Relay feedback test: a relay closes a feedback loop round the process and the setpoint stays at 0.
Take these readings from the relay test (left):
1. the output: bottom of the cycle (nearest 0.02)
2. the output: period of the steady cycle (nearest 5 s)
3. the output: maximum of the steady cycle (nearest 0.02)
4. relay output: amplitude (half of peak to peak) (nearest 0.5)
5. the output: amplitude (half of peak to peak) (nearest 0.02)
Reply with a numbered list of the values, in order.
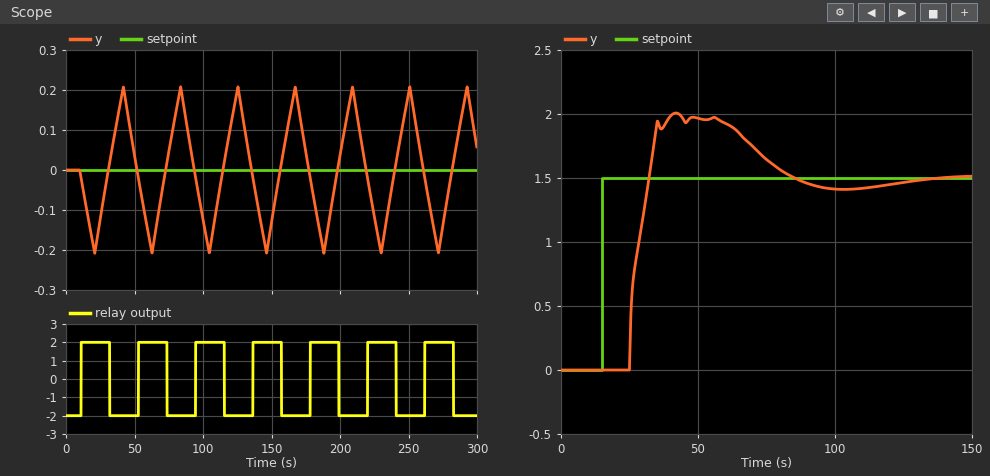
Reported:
1. -0.20
2. 40 s
3. 0.20
4. 2.0
5. 0.20
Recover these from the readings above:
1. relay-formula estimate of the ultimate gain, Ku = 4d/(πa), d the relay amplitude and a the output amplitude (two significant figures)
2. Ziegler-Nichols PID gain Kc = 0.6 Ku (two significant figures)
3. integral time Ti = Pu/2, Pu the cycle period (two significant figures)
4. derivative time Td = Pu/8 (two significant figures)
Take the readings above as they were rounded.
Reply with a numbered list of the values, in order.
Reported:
1. 13
2. 7.8
3. 20 s
4. 5.0 s
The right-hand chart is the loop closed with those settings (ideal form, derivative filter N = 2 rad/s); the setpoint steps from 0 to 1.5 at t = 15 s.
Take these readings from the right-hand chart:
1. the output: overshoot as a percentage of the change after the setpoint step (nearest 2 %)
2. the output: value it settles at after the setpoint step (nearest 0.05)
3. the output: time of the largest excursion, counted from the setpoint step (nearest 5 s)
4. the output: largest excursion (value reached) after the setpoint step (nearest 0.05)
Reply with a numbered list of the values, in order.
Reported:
1. 34 %
2. 1.50
3. 25 s
4. 2.00
